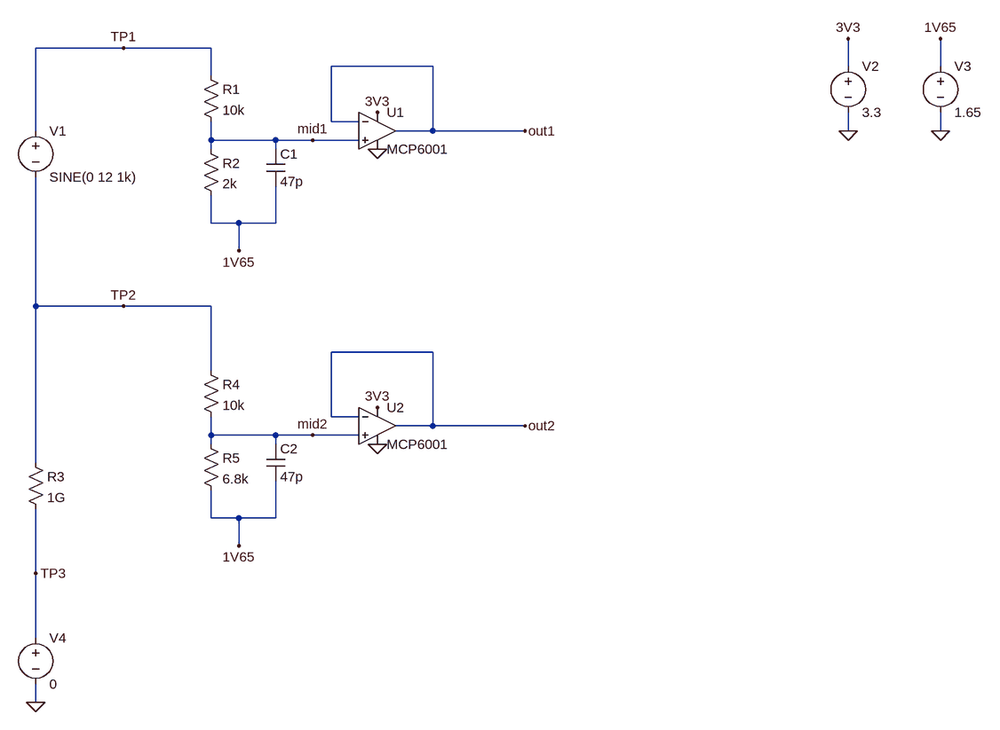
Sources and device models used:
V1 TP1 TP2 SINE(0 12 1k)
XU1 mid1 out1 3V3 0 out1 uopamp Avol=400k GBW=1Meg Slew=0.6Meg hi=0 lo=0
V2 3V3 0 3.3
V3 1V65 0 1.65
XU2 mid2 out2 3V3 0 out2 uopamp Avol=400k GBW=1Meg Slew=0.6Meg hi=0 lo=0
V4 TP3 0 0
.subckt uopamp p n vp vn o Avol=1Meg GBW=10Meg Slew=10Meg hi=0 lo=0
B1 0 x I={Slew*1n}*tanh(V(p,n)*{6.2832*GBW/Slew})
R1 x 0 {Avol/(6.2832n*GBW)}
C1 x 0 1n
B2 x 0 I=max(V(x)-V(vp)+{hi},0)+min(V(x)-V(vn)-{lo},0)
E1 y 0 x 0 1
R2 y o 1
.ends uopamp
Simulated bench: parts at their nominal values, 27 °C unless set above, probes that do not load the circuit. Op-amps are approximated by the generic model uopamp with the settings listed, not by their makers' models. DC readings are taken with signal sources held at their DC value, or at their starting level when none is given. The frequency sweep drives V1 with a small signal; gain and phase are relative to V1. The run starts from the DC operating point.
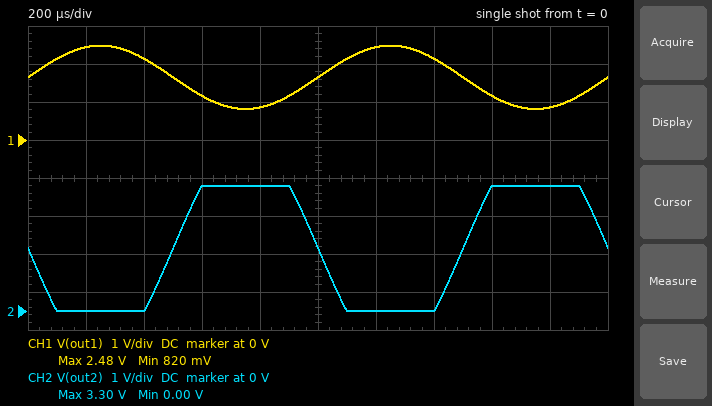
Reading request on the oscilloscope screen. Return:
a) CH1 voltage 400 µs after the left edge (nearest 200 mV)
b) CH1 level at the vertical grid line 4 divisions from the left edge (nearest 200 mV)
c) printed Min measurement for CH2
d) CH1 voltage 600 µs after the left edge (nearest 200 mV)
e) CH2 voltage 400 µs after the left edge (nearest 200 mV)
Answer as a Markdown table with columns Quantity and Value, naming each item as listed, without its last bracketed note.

| Quantity | Value |
|---|---|
| CH1 voltage 400 µs after the left edge | 2.2 V |
| CH1 level at the vertical grid line 4 divisions from the left edge | 800 mV |
| printed Min measurement for CH2 | 0.00 V |
| CH1 voltage 600 µs after the left edge | 1.2 V |
| CH2 voltage 400 µs after the left edge | 0 V |
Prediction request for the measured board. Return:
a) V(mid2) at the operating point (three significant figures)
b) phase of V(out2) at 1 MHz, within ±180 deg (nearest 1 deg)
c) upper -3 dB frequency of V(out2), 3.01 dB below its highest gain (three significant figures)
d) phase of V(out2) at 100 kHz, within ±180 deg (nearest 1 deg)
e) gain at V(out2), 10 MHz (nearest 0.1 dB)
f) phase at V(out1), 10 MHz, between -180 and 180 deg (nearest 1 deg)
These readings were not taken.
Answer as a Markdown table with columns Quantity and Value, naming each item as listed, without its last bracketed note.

| Quantity | Value |
|---|---|
| V(mid2) at the operating point | 1.65 V |
| phase of V(out2) at 1 MHz, within ±180 deg | 80 deg |
| upper -3 dB frequency of V(out2), 3.01 dB below its highest gain | 506 kHz |
| phase of V(out2) at 100 kHz, within ±180 deg | 166 deg |
| gain at V(out2), 10 MHz | -55.5 dB |
| phase at V(out1), 10 MHz, between -180 and 180 deg | -163 deg |
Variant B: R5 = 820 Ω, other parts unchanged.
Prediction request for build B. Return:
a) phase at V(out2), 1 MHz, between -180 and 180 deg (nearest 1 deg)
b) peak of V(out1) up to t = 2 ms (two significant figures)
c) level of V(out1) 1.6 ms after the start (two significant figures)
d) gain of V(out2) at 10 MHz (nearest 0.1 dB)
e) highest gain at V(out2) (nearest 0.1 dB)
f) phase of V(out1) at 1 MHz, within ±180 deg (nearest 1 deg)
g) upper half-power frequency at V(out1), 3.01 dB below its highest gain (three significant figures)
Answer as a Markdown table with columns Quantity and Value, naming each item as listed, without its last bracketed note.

| Quantity | Value |
|---|---|
| phase at V(out2), 1 MHz, between -180 and 180 deg | 124 deg |
| peak of V(out1) up to t = 2 ms | 2.7 V |
| level of V(out1) 1.6 ms after the start | 1.0 V |
| gain of V(out2) at 10 MHz | -56.2 dB |
| highest gain at V(out2) | -28.9 dB |
| phase of V(out1) at 1 MHz, within ±180 deg | -73 deg |
| upper half-power frequency at V(out1), 3.01 dB below its highest gain | 822 kHz |
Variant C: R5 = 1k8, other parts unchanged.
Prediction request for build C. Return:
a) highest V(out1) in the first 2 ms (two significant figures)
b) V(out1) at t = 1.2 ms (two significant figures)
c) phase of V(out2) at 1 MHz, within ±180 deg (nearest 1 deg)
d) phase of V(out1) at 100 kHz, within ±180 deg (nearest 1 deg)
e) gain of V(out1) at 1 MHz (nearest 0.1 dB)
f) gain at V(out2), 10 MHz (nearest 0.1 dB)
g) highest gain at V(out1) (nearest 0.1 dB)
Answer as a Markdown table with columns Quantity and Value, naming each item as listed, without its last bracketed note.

| Quantity | Value |
|---|---|
| highest V(out1) in the first 2 ms | 2.7 V |
| V(out1) at t = 1.2 ms | 2.6 V |
| phase of V(out2) at 1 MHz, within ±180 deg | 111 deg |
| phase of V(out1) at 100 kHz, within ±180 deg | -9 deg |
| gain of V(out1) at 1 MHz | -25.5 dB |
| gain at V(out2), 10 MHz | -55.7 dB |
| highest gain at V(out1) | -21.5 dB |
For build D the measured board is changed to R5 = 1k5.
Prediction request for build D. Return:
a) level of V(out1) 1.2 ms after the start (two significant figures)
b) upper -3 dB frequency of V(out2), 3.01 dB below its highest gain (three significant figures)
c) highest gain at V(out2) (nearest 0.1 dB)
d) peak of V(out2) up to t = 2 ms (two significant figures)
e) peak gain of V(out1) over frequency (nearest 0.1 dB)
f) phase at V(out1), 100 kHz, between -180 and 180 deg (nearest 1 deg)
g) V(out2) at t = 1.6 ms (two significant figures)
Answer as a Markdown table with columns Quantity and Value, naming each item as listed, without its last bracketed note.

| Quantity | Value |
|---|---|
| level of V(out1) 1.2 ms after the start | 2.6 V |
| upper -3 dB frequency of V(out2), 3.01 dB below its highest gain | 904 kHz |
| highest gain at V(out2) | -23.9 dB |
| peak of V(out2) up to t = 2 ms | 2.4 V |
| peak gain of V(out1) over frequency | -21.4 dB |
| phase at V(out1), 100 kHz, between -180 and 180 deg | -9 deg |
| V(out2) at t = 1.6 ms | 2.1 V |
